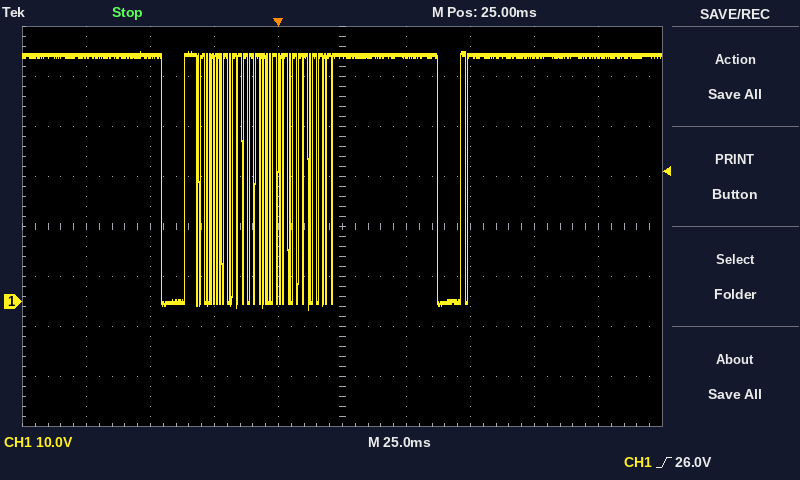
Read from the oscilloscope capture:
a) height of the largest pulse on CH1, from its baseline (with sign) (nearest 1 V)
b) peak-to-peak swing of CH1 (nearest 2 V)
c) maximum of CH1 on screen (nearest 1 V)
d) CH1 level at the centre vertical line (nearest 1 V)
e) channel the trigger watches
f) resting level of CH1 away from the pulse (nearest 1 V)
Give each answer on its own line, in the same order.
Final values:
-51 V
52 V
50 V
49 V
CH1
49 V
